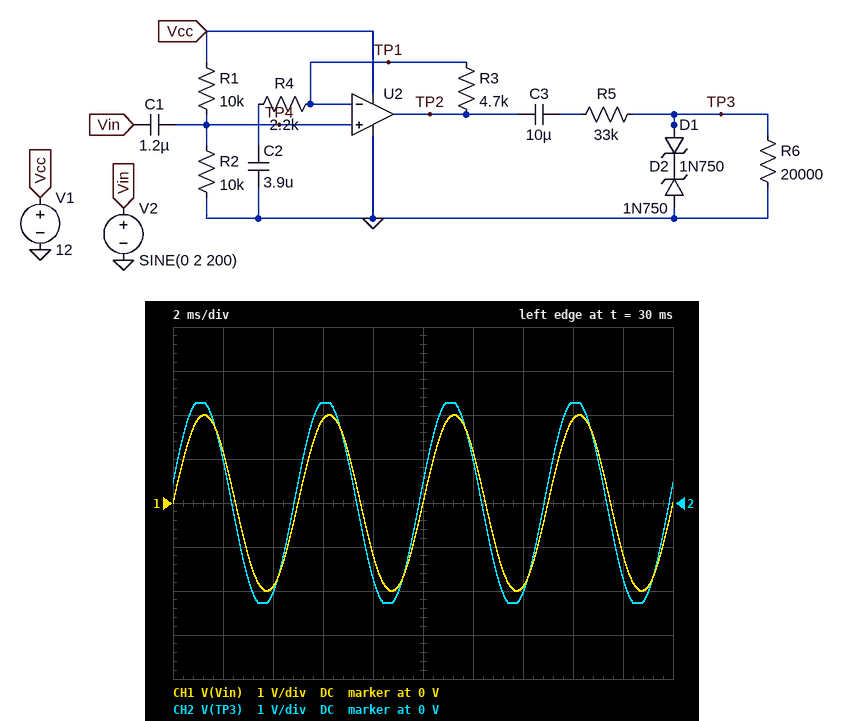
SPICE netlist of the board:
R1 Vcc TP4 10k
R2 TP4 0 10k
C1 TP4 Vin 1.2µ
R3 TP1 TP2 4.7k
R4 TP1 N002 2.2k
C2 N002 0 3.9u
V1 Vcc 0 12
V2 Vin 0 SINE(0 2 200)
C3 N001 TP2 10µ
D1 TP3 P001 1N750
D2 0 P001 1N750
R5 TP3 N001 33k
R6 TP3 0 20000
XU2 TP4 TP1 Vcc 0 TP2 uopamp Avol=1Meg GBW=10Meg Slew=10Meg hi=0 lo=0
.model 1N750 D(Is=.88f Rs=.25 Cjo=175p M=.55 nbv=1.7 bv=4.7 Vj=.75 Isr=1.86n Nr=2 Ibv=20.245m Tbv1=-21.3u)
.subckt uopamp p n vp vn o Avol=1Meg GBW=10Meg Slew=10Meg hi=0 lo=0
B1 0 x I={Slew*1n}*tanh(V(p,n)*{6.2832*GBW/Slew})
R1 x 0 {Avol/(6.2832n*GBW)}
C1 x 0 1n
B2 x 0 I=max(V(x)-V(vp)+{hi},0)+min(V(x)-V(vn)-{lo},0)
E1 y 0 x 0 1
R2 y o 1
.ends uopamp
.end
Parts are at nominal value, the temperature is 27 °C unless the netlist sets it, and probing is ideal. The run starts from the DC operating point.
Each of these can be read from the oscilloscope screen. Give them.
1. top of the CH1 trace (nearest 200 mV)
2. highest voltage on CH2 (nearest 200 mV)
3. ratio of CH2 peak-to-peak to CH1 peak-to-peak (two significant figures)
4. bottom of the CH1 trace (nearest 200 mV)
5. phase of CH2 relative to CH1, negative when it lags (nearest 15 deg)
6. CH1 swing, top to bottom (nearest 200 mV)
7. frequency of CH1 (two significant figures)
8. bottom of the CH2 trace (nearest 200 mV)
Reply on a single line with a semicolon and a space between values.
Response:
2.0 V; 2.2 V; 1.1; -2.0 V; 15 deg; 4.0 V; 200 Hz; -2.2 V
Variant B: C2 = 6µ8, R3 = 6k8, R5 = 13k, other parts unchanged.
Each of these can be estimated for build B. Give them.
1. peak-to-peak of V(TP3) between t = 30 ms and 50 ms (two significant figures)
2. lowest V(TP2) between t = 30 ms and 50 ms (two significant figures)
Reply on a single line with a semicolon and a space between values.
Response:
7.3 V; -9.1 mV
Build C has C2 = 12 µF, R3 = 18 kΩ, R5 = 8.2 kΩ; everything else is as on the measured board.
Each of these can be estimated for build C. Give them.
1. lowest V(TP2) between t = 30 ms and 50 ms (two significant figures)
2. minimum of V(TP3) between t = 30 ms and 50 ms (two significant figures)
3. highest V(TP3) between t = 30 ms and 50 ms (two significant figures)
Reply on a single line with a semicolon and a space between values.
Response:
-9.5 mV; -4.3 V; 4.3 V
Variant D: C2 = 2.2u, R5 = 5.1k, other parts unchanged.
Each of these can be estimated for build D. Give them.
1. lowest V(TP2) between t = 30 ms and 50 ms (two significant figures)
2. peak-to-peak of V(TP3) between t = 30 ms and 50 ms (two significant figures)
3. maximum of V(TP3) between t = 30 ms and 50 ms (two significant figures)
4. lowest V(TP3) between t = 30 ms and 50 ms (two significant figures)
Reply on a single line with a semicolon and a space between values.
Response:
-1.7 mV; 9.5 V; 4.8 V; -4.8 V
